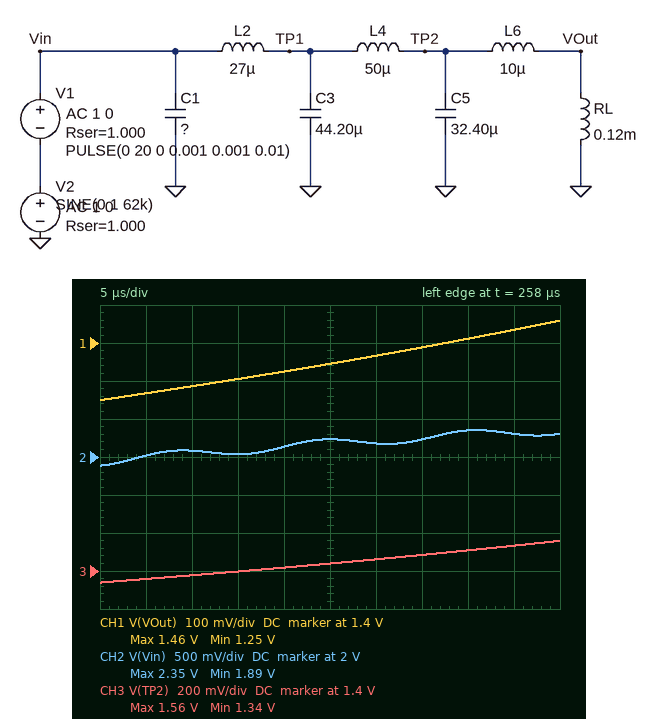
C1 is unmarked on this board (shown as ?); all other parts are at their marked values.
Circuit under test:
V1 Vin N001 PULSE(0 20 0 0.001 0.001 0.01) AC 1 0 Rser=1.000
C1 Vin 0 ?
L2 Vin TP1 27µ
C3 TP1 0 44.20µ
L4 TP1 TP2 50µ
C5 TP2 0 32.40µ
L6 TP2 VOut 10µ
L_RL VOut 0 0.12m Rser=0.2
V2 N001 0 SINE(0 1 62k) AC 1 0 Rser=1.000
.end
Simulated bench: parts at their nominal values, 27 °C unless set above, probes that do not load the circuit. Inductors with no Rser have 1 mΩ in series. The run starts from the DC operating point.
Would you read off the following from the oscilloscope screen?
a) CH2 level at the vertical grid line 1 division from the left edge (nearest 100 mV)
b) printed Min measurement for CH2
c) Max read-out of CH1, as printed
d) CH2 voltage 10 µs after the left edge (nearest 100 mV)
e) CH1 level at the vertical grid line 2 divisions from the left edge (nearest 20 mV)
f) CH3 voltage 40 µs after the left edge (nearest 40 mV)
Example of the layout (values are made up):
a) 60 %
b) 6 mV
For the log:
a) 2.0 V
b) 1.89 V
c) 1.46 V
d) 2.1 V
e) 1.28 V
f) 1.52 V
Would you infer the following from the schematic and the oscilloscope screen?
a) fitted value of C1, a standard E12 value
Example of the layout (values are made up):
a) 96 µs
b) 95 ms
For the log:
a) 22 µF
